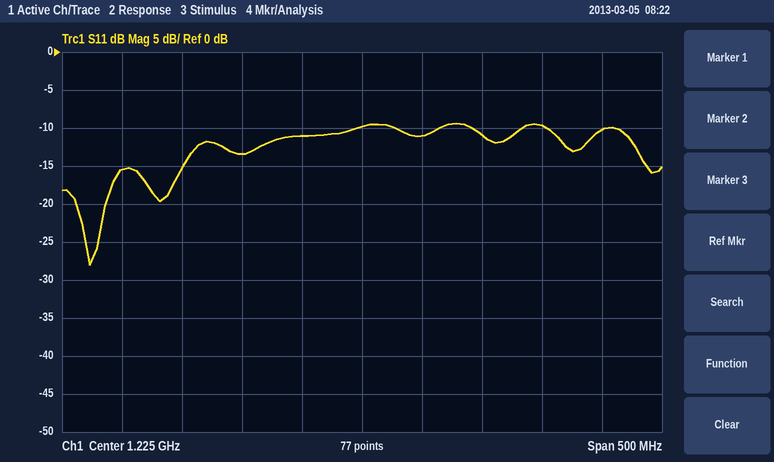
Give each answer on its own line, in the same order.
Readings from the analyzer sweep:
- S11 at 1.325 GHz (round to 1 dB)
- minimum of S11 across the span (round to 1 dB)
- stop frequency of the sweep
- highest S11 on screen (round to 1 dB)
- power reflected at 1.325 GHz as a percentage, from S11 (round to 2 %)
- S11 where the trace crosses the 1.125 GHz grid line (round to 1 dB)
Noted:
-11 dB
-28 dB
1.475 GHz
-9 dB
8 %
-13 dB
